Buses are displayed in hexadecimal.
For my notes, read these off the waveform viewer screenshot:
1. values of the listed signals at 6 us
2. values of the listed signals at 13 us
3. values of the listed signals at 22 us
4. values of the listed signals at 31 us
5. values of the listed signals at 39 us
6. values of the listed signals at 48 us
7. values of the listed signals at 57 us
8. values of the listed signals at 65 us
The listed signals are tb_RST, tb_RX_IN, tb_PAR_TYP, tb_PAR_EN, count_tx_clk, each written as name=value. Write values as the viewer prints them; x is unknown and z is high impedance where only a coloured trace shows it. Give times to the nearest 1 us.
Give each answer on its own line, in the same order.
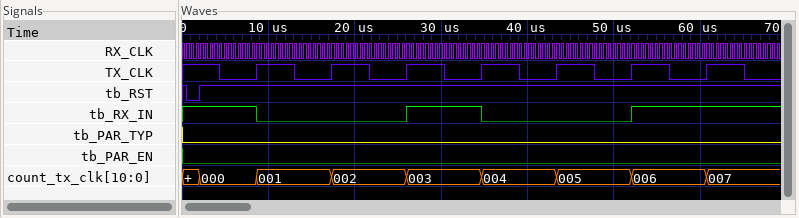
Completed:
tb_RST=1, tb_RX_IN=1, tb_PAR_TYP=0, tb_PAR_EN=0, count_tx_clk=000
tb_RST=1, tb_RX_IN=0, tb_PAR_TYP=0, tb_PAR_EN=0, count_tx_clk=001
tb_RST=1, tb_RX_IN=0, tb_PAR_TYP=0, tb_PAR_EN=0, count_tx_clk=002
tb_RST=1, tb_RX_IN=1, tb_PAR_TYP=0, tb_PAR_EN=0, count_tx_clk=003
tb_RST=1, tb_RX_IN=0, tb_PAR_TYP=0, tb_PAR_EN=0, count_tx_clk=004
tb_RST=1, tb_RX_IN=0, tb_PAR_TYP=0, tb_PAR_EN=0, count_tx_clk=005
tb_RST=1, tb_RX_IN=1, tb_PAR_TYP=0, tb_PAR_EN=0, count_tx_clk=006
tb_RST=1, tb_RX_IN=1, tb_PAR_TYP=0, tb_PAR_EN=0, count_tx_clk=007
